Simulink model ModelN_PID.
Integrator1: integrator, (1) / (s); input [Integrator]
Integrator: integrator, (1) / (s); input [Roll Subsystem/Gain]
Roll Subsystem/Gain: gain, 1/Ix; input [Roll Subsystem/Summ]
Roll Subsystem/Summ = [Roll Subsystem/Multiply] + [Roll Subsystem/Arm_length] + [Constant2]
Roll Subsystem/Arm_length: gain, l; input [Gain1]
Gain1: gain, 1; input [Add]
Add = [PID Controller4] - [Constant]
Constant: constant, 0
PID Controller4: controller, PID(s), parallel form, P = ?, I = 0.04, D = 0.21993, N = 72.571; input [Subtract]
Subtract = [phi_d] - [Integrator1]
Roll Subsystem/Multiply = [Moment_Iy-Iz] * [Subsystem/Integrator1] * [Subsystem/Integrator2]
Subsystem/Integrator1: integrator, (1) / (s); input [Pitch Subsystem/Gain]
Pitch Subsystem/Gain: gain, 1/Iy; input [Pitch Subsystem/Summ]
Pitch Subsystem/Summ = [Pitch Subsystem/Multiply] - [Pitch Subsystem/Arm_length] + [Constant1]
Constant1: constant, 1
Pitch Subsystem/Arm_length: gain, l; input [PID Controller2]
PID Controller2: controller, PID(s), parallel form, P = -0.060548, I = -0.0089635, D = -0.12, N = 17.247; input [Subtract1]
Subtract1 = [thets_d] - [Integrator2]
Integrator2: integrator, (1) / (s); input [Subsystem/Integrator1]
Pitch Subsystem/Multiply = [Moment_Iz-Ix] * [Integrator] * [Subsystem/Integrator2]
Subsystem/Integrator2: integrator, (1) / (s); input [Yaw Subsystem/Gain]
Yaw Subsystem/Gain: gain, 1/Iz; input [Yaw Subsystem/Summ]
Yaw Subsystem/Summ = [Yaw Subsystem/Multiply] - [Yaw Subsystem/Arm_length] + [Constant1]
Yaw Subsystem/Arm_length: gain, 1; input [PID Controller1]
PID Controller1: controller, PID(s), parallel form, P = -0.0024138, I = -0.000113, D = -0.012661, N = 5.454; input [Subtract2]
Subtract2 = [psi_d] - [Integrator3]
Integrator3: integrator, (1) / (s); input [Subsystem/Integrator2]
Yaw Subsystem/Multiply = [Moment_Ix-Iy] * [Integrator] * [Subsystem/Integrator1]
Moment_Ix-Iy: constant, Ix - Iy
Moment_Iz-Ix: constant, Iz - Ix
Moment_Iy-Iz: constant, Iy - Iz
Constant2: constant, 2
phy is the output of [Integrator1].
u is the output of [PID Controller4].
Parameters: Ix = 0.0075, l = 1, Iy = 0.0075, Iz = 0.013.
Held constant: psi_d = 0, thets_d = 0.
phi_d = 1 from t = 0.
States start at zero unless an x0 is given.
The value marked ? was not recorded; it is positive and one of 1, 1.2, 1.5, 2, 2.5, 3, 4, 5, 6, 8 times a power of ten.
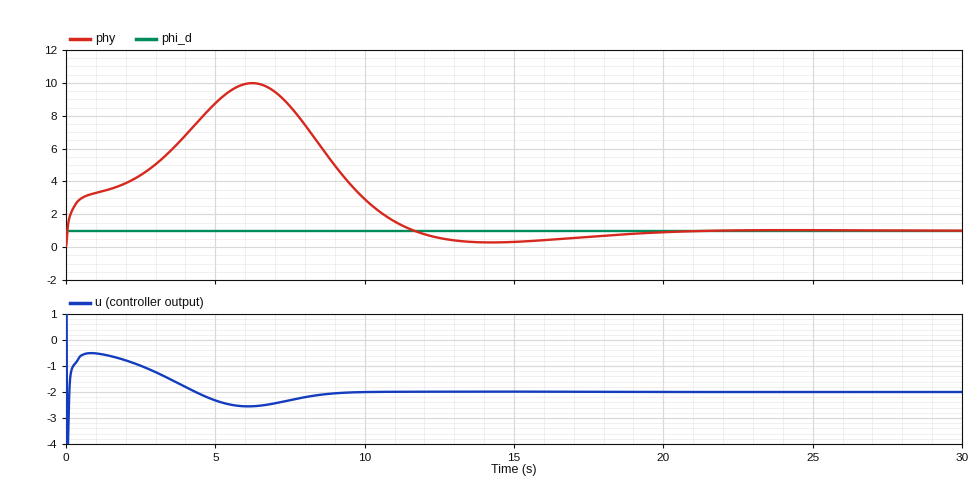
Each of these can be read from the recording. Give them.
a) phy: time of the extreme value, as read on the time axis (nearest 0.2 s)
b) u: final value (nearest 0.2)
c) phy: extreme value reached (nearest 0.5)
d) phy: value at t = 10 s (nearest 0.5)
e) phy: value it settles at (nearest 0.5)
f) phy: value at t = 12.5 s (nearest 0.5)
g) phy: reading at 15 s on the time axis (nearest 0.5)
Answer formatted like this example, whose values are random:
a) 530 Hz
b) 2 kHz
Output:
a) 6.2 s
b) -2.0
c) 10.0
d) 3.0
e) 1.0
f) 0.5
g) 0.5
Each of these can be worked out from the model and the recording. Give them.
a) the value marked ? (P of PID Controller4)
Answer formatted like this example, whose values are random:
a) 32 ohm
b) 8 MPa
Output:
a) 0.15
